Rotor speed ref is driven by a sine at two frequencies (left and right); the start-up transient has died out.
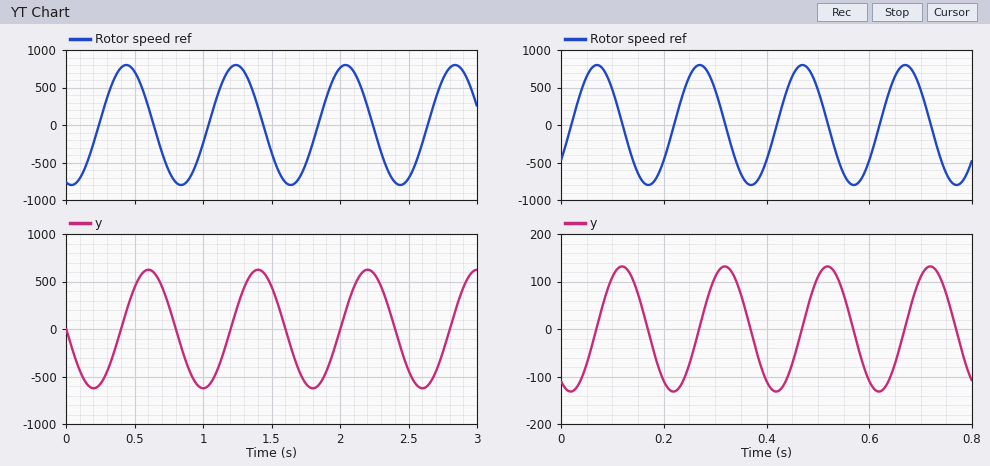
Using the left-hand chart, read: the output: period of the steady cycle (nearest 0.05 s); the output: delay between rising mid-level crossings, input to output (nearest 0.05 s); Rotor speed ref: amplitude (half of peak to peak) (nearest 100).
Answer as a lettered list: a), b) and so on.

a) 0.80 s
b) 0.15 s
c) 800
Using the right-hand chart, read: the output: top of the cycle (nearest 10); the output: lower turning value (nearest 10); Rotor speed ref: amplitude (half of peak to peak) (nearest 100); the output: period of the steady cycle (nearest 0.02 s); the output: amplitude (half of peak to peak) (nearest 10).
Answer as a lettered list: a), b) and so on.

a) 130
b) -130
c) 800
d) 0.20 s
e) 130
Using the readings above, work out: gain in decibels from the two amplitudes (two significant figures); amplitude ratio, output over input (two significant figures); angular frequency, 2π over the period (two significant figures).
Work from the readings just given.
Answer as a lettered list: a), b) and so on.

a) -16 dB
b) 0.16
c) 31 rad/s
